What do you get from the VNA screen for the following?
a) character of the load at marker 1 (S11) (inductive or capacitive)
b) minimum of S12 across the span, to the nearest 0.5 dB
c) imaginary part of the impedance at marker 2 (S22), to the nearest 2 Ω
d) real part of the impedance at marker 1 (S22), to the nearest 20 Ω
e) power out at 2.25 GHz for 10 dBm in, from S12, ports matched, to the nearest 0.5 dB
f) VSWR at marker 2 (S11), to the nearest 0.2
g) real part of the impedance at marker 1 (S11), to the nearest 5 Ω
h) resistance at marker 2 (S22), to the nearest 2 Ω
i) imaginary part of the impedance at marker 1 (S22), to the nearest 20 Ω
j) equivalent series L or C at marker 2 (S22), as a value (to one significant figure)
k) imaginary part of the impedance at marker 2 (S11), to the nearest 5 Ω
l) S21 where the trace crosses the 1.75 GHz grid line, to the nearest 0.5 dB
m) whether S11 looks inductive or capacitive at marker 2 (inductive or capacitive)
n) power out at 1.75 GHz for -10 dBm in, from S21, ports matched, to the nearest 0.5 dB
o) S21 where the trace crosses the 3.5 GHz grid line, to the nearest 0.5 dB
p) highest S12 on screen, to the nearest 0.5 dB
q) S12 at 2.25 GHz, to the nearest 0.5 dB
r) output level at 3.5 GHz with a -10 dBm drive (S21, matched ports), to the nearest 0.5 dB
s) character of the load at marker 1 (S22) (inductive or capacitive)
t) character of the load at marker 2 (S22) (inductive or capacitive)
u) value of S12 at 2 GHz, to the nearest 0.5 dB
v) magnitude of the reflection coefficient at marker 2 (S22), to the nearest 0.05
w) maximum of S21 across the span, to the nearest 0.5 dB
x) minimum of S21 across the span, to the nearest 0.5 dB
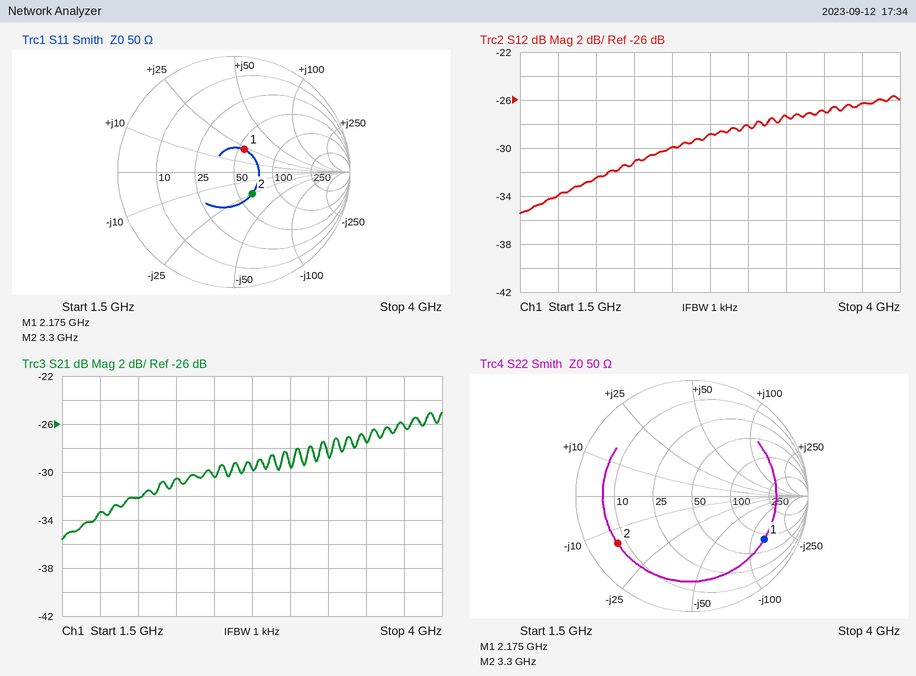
inductive
-35.5 dB
-14 Ω
80 Ω
-21.0 dBm
1.6
55 Ω
8 Ω
-140 Ω
3 pF
-25 Ω
-33.5 dB
capacitive
-43.5 dBm
-27.5 dB
-25.5 dB
-31.0 dB
-37.5 dBm
capacitive
capacitive
-32.5 dB
0.75
-25.0 dB
-35.5 dB
